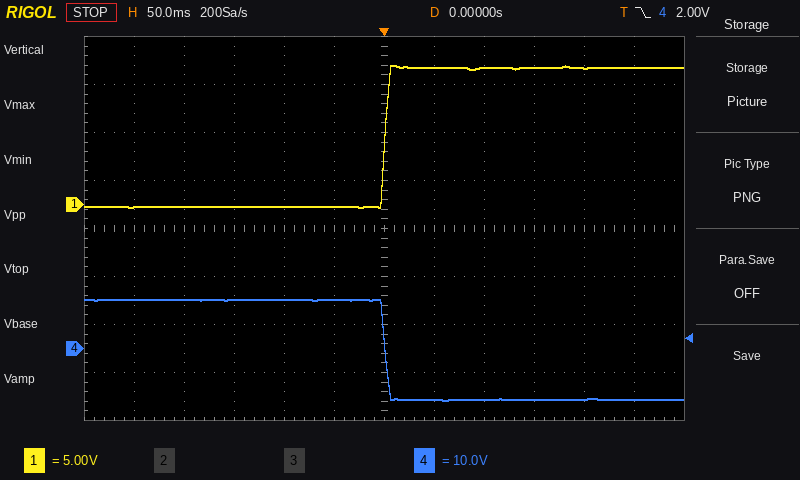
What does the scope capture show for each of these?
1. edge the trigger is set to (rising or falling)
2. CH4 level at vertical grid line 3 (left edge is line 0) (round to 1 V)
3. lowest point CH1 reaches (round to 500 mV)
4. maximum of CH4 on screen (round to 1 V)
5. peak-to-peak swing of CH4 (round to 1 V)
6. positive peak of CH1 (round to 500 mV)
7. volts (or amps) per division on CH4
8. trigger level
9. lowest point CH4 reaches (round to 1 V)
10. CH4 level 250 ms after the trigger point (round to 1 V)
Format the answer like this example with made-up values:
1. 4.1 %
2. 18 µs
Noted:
1. falling
2. 10 V
3. -500 mV
4. 10 V
5. 21 V
6. 14.5 V
7. 10 V
8. 2.00 V
9. -11 V
10. -11 V
